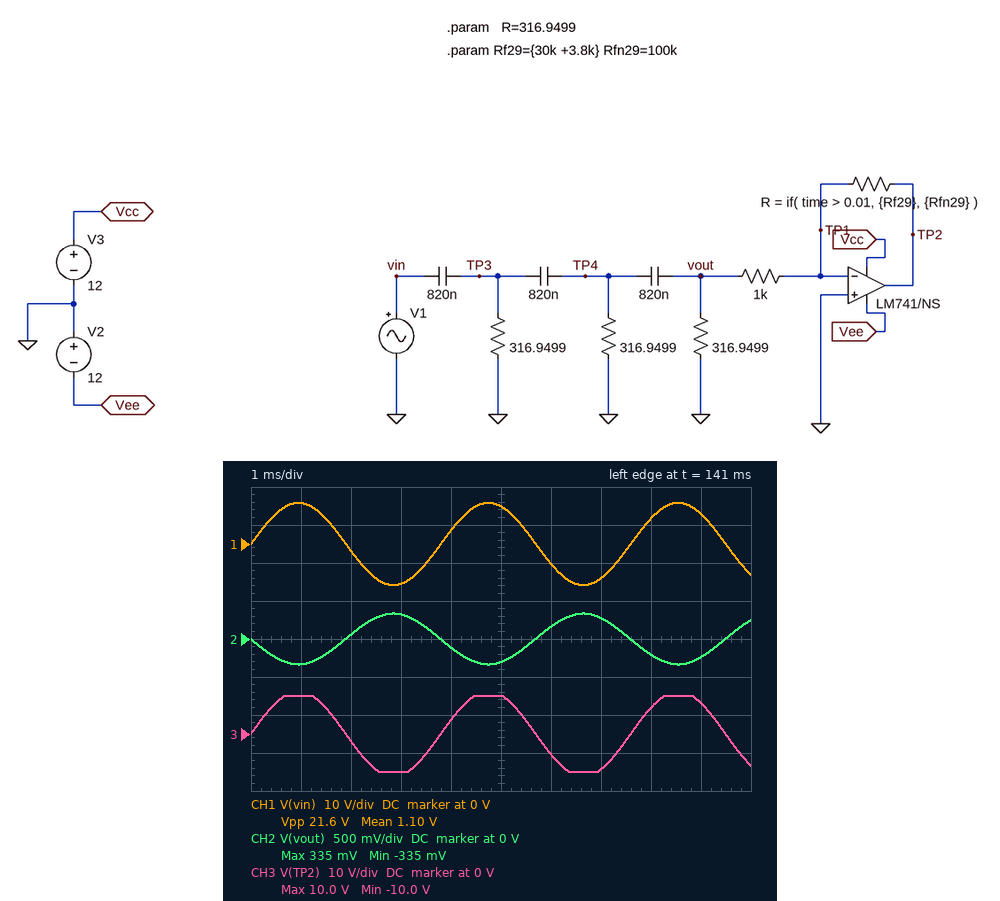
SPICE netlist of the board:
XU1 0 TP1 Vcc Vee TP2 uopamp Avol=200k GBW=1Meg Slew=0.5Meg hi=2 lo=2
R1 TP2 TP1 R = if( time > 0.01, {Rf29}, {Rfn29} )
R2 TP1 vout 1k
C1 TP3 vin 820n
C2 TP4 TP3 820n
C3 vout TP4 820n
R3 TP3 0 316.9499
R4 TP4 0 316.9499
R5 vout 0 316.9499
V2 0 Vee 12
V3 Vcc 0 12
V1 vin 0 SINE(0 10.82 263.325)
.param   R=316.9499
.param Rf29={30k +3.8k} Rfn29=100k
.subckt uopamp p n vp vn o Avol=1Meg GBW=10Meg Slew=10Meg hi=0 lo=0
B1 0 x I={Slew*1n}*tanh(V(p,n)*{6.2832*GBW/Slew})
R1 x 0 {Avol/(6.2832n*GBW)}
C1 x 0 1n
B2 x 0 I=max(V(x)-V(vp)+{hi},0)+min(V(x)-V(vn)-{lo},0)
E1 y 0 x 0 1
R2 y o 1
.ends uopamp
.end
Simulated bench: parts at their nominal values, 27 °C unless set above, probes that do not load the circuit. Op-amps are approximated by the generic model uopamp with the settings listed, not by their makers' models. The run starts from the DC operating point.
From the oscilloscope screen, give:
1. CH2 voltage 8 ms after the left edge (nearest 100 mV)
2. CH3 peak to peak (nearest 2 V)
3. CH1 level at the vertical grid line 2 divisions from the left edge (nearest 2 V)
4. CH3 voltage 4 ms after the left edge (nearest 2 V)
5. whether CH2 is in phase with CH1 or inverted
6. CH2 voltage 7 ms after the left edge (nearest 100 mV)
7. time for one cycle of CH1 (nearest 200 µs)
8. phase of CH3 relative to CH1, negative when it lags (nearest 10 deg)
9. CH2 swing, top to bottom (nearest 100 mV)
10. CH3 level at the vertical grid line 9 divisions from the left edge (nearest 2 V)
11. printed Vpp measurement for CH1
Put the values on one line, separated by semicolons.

-200 mV; 20 V; -2 V; 4 V; inverted; 300 mV; 3.8 ms; 0 deg; 700 mV; 8 V; 21.6 V
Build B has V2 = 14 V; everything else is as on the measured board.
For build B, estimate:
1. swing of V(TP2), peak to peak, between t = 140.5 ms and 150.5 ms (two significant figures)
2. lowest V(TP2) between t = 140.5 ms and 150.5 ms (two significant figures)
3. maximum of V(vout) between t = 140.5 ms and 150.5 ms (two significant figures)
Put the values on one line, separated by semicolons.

21 V; -11 V; 330 mV
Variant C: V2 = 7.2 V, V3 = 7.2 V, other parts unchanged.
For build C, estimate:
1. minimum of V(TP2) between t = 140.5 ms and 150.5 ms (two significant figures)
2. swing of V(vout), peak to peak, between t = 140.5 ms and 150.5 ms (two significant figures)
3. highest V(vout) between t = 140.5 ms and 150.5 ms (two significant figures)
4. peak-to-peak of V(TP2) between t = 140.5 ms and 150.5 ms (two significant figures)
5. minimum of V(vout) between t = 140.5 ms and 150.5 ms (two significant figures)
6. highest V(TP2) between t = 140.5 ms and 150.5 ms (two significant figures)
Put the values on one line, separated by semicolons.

-5.2 V; 740 mV; 370 mV; 10 V; -370 mV; 5.2 V
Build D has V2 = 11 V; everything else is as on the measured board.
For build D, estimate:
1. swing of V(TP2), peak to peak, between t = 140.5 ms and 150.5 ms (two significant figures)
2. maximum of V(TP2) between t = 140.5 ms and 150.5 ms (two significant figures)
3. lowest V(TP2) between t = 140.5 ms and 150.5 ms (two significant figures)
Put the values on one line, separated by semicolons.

19 V; 10 V; -9.0 V
